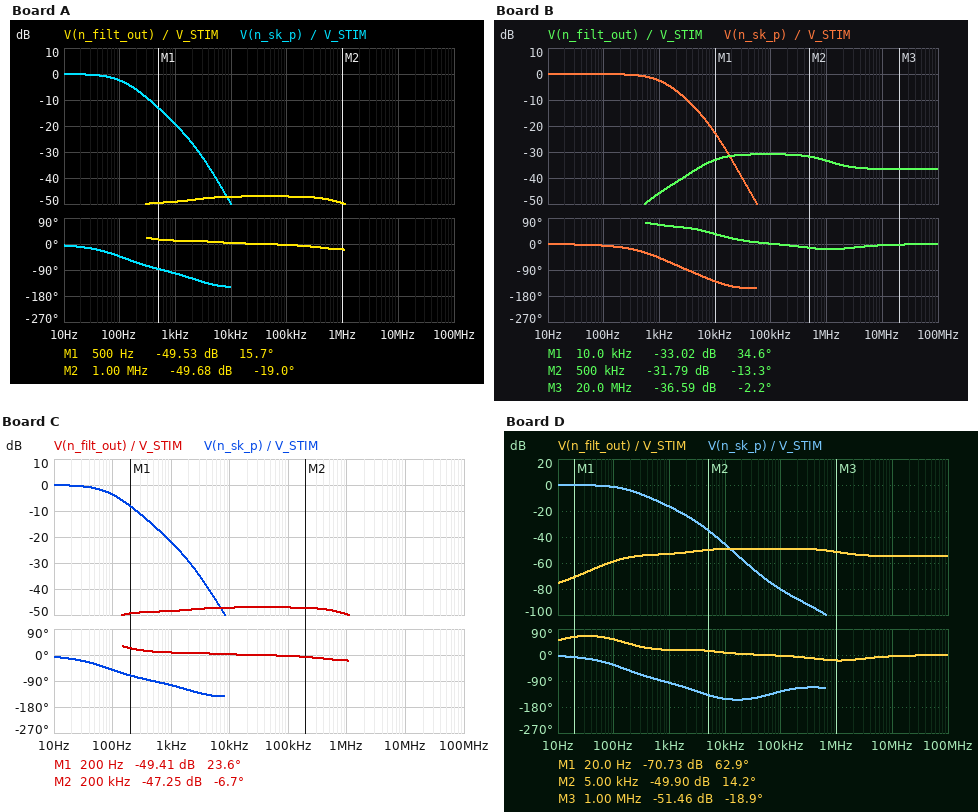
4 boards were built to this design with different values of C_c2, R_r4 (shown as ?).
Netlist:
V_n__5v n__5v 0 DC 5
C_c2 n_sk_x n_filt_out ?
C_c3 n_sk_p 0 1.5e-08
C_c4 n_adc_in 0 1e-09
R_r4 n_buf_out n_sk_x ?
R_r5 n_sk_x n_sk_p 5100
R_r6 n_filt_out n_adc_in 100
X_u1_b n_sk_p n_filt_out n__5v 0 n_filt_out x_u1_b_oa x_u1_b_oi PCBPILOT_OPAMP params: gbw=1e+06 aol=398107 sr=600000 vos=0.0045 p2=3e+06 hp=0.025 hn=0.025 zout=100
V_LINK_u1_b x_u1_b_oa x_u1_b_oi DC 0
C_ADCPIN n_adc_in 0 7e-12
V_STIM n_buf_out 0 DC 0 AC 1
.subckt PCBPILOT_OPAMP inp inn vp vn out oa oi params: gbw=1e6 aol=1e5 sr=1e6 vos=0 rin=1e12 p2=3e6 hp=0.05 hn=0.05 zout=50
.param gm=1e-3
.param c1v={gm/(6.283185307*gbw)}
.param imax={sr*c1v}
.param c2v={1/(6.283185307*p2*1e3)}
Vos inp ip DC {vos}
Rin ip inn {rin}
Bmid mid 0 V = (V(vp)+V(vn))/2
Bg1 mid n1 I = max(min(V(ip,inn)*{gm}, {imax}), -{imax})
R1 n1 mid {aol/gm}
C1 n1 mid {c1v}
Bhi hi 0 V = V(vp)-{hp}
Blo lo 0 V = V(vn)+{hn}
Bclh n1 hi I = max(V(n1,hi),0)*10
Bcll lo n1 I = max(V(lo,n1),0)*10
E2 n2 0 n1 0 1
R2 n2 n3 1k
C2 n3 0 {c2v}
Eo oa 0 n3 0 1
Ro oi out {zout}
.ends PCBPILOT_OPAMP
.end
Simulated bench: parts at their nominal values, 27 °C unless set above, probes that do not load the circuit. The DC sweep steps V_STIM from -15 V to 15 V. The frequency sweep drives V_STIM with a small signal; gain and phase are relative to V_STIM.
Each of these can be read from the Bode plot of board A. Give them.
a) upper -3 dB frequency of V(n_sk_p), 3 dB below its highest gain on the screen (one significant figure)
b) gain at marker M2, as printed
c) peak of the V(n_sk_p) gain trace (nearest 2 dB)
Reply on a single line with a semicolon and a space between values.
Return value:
100 Hz; -49.68 dB; 0 dB
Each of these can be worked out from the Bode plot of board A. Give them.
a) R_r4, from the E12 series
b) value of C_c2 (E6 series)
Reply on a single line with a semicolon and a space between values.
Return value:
22 kΩ; 47 nF
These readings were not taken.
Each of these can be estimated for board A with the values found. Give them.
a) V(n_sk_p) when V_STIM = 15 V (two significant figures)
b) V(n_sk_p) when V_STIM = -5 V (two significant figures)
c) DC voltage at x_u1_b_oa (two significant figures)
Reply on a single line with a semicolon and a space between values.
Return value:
15 V; -5.0 V; 25 mV
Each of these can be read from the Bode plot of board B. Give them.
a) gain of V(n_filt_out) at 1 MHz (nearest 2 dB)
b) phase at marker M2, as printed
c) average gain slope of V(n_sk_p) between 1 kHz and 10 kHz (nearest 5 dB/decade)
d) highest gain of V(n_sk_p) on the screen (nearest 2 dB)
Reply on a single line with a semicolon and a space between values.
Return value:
-34 dB; -13.3 deg; -20 dB/decade; 0 dB
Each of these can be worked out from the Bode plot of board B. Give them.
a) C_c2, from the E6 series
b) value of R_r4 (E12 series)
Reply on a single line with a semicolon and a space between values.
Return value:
10 nF; 3.3 kΩ
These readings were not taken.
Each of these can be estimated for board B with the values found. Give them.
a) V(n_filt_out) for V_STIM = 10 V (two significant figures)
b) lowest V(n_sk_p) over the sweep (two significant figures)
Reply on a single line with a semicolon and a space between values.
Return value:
5.0 V; -15 V
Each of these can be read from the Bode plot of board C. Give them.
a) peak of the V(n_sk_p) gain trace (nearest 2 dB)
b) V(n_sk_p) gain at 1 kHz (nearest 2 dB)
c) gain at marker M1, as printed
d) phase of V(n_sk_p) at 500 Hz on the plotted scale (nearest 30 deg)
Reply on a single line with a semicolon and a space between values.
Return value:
0 dB; -22 dB; -49.41 dB; -90 deg
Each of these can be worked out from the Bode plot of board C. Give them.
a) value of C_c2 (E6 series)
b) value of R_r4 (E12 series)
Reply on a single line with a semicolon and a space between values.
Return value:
68 nF; 22 kΩ
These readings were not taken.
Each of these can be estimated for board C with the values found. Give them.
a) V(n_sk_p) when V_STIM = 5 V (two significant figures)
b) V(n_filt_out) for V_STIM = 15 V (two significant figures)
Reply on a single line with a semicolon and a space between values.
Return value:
5.0 V; 5.0 V
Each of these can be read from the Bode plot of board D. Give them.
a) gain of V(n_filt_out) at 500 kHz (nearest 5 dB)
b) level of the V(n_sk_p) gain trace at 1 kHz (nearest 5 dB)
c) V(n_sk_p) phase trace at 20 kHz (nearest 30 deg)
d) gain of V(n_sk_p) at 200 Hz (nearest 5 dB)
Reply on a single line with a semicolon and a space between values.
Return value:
-50 dB; -15 dB; -150 deg; -5 dB
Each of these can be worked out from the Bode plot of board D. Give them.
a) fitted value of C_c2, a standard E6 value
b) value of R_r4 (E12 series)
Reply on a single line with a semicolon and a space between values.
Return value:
22 nF; 27 kΩ
